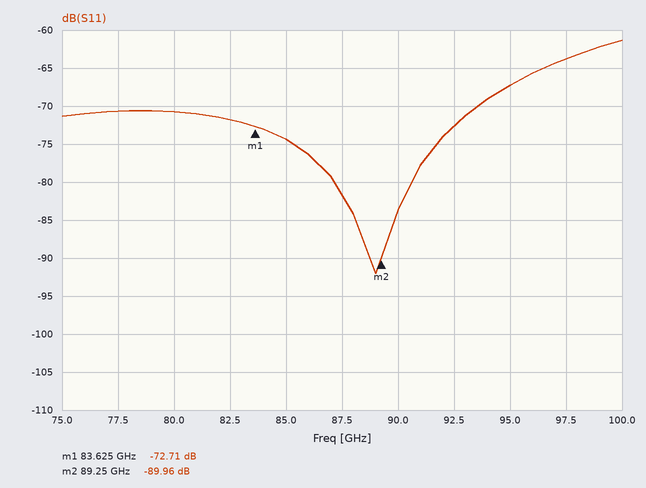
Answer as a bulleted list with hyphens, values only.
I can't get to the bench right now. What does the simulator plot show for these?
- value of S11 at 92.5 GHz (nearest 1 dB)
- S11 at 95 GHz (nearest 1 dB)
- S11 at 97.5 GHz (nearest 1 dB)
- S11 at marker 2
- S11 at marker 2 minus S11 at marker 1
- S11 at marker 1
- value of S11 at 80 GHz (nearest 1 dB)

- -73 dB
- -67 dB
- -64 dB
- -89.96 dB
- -17.25 dB
- -72.71 dB
- -71 dB
